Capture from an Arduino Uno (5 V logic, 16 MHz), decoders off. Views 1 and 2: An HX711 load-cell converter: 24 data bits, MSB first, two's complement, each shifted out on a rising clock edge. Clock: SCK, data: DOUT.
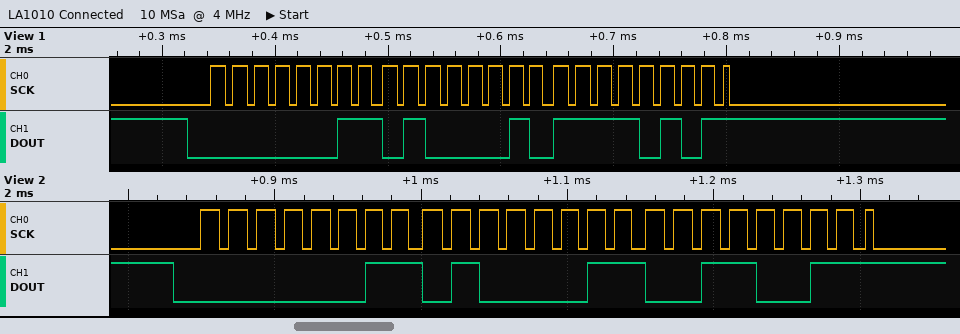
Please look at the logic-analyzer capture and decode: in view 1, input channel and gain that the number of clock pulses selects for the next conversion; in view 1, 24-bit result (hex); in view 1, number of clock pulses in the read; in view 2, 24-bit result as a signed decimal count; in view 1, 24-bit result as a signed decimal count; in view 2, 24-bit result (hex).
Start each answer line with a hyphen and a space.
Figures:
- channel A, gain 128
- 0x0342F5
- 25
- 213811
- 213749
- 0x034333
